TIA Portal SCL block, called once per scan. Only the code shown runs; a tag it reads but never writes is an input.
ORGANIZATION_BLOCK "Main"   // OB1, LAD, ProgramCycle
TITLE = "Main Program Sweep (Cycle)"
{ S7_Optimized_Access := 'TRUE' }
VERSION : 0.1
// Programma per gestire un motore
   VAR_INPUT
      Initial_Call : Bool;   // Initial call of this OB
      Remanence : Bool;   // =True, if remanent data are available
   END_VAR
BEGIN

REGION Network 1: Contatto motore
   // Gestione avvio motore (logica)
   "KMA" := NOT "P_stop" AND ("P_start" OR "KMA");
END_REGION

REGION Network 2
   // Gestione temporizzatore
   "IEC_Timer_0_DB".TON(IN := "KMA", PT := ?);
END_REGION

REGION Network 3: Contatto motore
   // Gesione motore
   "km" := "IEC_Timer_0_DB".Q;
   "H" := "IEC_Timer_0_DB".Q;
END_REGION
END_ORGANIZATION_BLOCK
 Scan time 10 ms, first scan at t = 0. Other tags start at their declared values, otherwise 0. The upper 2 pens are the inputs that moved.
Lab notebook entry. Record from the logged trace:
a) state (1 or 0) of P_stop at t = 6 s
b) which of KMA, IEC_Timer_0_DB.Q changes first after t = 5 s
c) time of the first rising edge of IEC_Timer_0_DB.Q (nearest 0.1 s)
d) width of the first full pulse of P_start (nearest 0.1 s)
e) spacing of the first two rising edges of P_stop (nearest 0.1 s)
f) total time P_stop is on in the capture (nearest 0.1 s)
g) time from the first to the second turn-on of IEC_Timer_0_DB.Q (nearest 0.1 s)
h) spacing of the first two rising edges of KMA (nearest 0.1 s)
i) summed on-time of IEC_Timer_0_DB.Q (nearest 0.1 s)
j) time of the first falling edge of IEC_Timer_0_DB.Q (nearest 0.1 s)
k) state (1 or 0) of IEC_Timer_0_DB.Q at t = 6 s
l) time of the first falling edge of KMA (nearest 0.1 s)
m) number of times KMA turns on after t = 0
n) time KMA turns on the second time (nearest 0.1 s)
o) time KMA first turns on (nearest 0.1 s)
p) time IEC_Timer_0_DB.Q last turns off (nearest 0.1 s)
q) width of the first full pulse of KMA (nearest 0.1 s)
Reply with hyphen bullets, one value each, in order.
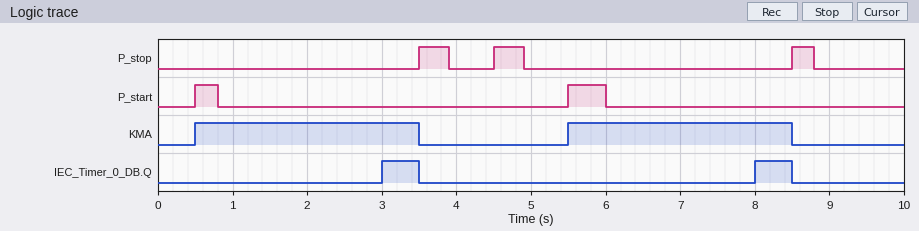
- 0
- KMA
- 3.0 s
- 0.3 s
- 1.0 s
- 1.1 s
- 5.0 s
- 5.0 s
- 1.0 s
- 3.5 s
- 0
- 3.5 s
- 2
- 5.5 s
- 0.5 s
- 8.5 s
- 3.0 s
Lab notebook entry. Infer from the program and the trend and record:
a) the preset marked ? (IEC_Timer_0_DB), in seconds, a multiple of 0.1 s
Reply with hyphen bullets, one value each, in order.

- 2.5 s
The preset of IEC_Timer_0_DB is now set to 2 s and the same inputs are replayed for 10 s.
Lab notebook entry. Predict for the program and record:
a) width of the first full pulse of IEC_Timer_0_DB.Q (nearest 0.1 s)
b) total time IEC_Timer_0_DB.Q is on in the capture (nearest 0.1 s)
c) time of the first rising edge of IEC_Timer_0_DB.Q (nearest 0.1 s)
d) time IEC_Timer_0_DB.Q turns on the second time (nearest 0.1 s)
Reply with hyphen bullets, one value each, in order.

- 1.0 s
- 2.0 s
- 2.5 s
- 7.5 s
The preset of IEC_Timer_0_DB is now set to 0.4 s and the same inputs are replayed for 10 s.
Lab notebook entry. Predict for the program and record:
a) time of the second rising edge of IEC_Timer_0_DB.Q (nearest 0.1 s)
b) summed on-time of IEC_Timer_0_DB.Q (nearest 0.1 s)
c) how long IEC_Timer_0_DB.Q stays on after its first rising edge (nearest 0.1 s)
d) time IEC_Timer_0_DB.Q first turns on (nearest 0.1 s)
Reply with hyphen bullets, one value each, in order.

- 5.9 s
- 5.2 s
- 2.6 s
- 0.9 s
